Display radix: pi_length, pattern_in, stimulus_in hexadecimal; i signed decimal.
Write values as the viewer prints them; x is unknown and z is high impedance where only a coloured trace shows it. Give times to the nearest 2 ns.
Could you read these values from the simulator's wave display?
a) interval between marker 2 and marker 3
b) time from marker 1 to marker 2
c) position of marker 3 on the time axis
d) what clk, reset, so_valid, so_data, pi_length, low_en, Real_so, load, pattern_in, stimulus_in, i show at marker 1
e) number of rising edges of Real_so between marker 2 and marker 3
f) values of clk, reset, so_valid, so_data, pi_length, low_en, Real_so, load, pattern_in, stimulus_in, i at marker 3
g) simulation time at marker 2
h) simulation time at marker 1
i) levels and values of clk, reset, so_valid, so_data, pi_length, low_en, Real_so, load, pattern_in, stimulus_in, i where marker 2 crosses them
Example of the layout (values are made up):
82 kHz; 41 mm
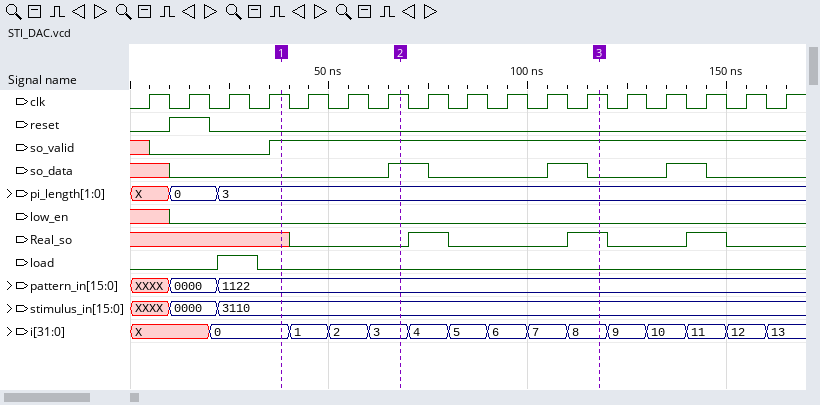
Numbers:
50 ns; 30 ns; 118 ns; clk=1, reset=0, so_valid=1, so_data=0, pi_length=3, low_en=0, Real_so=x, load=0, pattern_in=1122, stimulus_in=3110, i=0; 2; clk=1, reset=0, so_valid=1, so_data=0, pi_length=3, low_en=0, Real_so=1, load=0, pattern_in=1122, stimulus_in=3110, i=8; 68 ns; 38 ns; clk=1, reset=0, so_valid=1, so_data=1, pi_length=3, low_en=0, Real_so=0, load=0, pattern_in=1122, stimulus_in=3110, i=3
